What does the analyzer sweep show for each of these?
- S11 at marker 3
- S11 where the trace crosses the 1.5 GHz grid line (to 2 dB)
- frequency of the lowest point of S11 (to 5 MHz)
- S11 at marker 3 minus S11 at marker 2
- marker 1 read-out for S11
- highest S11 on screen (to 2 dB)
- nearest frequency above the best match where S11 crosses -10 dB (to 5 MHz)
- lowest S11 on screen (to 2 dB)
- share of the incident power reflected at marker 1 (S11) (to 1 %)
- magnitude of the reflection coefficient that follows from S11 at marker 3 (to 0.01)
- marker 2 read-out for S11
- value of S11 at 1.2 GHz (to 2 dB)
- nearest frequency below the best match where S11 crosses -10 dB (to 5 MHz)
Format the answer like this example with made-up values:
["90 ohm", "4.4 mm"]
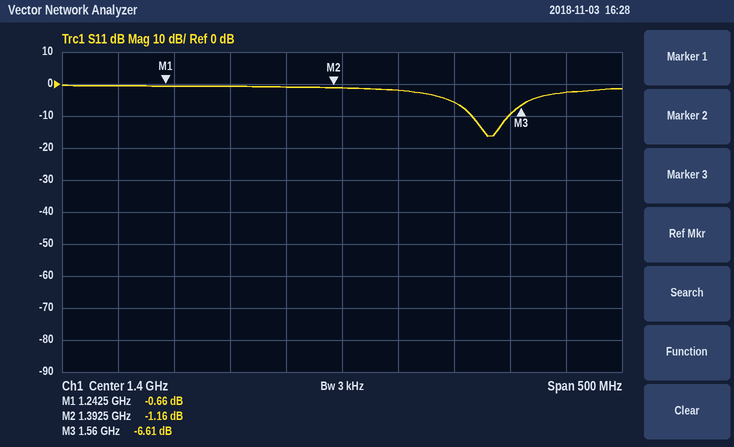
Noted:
["-6.61 dB", "-6 dB", "1.530 GHz", "-5.45 dB", "-0.66 dB", "0 dB", "1.550 GHz", "-16 dB", "86 %", "0.47", "-1.16 dB", "0 dB", "1.515 GHz"]
